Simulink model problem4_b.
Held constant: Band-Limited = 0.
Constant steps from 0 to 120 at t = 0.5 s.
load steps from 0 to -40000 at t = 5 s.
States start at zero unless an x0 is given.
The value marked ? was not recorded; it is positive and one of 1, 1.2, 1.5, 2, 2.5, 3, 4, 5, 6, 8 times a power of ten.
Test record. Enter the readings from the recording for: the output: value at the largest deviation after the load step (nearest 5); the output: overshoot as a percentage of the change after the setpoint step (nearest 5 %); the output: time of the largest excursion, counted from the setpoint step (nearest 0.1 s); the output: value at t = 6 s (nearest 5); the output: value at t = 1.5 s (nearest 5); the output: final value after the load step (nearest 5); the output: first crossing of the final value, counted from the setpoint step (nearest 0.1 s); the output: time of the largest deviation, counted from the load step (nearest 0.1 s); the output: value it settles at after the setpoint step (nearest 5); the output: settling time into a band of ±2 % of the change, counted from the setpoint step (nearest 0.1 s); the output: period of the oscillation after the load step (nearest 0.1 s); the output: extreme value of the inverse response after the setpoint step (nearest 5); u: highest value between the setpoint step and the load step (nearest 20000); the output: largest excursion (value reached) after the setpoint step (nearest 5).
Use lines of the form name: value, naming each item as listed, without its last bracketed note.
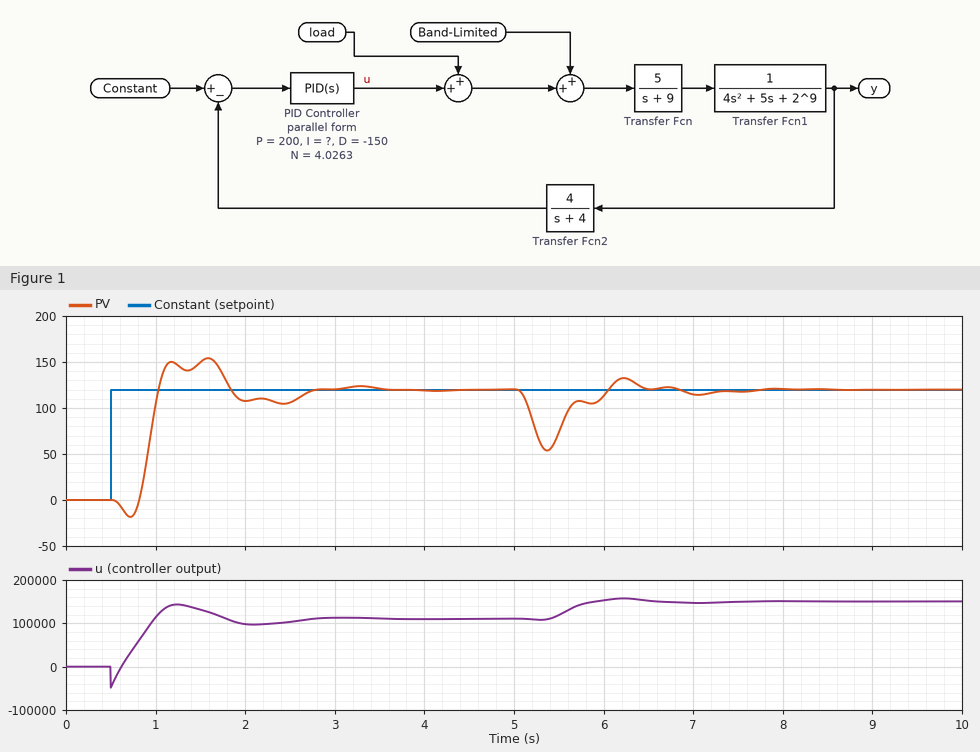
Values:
the output: value at the largest deviation after the load step: 55
the output: overshoot as a percentage of the change after the setpoint step: 30 %
the output: time of the largest excursion, counted from the setpoint step: 1.1 s
the output: value at t = 6 s: 115
the output: value at t = 1.5 s: 150
the output: final value after the load step: 120
the output: first crossing of the final value, counted from the setpoint step: 0.5 s
the output: time of the largest deviation, counted from the load step: 0.4 s
the output: value it settles at after the setpoint step: 120
the output: settling time into a band of ±2 % of the change, counted from the setpoint step: 2.9 s
the output: period of the oscillation after the load step: 1.7 s
the output: extreme value of the inverse response after the setpoint step: -20
u: highest value between the setpoint step and the load step: 140000
the output: largest excursion (value reached) after the setpoint step: 155
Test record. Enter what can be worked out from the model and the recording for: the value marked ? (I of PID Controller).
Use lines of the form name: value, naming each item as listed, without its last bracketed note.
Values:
the value marked ?: 1500
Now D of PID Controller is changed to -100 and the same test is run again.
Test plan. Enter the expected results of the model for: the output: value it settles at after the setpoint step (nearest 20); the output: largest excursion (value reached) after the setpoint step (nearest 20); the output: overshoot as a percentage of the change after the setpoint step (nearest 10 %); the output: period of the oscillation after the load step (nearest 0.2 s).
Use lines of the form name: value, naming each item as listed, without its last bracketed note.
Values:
the output: value it settles at after the setpoint step: 120
the output: largest excursion (value reached) after the setpoint step: 140
the output: overshoot as a percentage of the change after the setpoint step: 20 %
the output: period of the oscillation after the load step: 0.6 s
